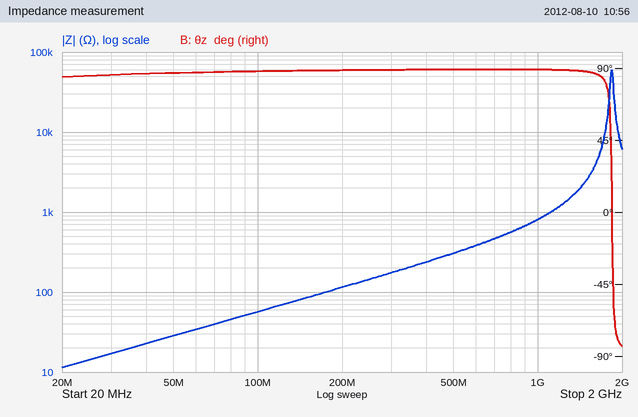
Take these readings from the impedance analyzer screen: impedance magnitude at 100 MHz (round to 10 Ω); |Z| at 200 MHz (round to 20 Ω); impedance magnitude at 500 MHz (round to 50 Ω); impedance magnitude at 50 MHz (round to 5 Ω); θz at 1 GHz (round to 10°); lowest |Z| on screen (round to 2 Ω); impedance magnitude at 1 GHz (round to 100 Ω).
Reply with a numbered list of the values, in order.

1. 60 Ω
2. 120 Ω
3. 300 Ω
4. 30 Ω
5. 90°
6. 12 Ω
7. 800 Ω
